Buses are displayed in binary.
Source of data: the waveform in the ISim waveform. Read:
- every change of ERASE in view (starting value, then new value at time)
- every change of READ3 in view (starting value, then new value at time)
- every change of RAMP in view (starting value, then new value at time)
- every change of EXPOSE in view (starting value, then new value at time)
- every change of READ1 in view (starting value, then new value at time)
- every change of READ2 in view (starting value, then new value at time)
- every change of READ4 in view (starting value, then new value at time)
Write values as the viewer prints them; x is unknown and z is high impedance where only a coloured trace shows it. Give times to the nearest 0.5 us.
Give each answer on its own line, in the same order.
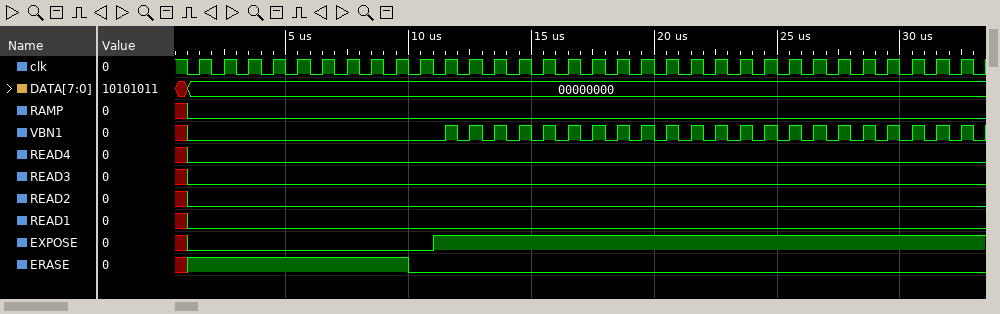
x, 1 at 1 us, 0 at 10 us
x, 0 at 1 us
x, 0 at 1 us
x, 0 at 1 us, 1 at 11 us
x, 0 at 1 us
x, 0 at 1 us
x, 0 at 1 us
